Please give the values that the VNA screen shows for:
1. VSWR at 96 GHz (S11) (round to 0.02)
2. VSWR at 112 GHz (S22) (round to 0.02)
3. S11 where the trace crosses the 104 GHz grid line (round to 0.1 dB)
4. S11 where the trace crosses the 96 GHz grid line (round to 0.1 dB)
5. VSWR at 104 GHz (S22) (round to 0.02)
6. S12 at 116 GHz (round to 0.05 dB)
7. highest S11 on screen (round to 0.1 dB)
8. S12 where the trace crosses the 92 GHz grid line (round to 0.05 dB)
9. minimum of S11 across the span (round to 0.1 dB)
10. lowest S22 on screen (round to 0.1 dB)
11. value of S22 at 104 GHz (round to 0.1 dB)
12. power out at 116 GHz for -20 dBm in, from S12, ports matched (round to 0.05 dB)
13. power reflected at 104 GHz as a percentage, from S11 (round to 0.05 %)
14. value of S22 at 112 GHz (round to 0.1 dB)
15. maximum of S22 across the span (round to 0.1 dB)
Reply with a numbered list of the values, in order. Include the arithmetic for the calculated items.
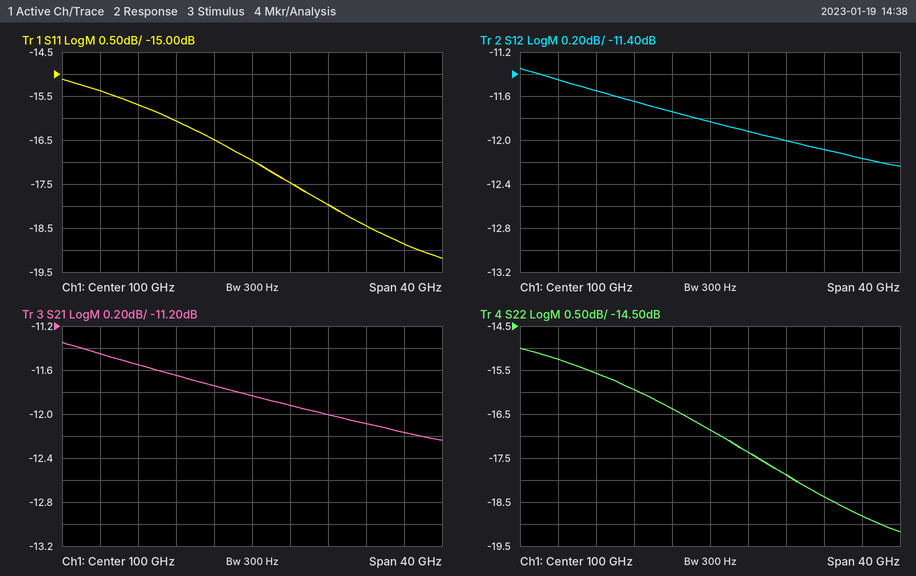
1. |Γ| = 10^(-16.5/20) = 0.1496; VSWR = (1 + 0.1496)/(1 − 0.1496) ≈ 1.35, so 1.36 to the nearest 0.02
2. |Γ| = 10^(-18.4/20) = 0.1202; VSWR = (1 + 0.1202)/(1 − 0.1202) ≈ 1.27, so 1.28 to the nearest 0.02
3. -17.5 dB
4. -16.5 dB
5. |Γ| = 10^(-17.4/20) = 0.1349; VSWR = (1 + 0.1349)/(1 − 0.1349) ≈ 1.31, so 1.32 to the nearest 0.02
6. -12.15 dB
7. -15.1 dB
8. -11.65 dB
9. -19.2 dB
10. -19.2 dB
11. -17.4 dB
12. -20 dBm + (-12.15 dB) = -32.15 dBm
13. 10^(-17.5/10) ≈ 1.78 %, so 1.80 % to the nearest 0.05 %
14. -18.4 dB
15. -15.0 dB
